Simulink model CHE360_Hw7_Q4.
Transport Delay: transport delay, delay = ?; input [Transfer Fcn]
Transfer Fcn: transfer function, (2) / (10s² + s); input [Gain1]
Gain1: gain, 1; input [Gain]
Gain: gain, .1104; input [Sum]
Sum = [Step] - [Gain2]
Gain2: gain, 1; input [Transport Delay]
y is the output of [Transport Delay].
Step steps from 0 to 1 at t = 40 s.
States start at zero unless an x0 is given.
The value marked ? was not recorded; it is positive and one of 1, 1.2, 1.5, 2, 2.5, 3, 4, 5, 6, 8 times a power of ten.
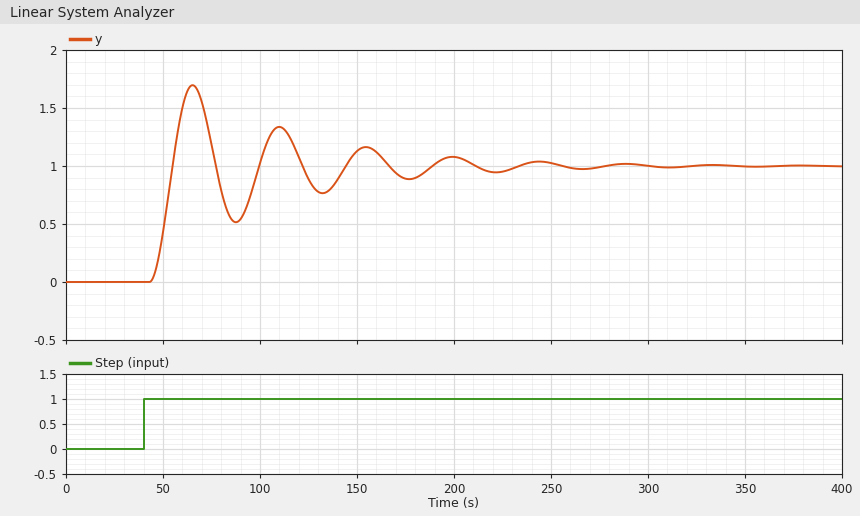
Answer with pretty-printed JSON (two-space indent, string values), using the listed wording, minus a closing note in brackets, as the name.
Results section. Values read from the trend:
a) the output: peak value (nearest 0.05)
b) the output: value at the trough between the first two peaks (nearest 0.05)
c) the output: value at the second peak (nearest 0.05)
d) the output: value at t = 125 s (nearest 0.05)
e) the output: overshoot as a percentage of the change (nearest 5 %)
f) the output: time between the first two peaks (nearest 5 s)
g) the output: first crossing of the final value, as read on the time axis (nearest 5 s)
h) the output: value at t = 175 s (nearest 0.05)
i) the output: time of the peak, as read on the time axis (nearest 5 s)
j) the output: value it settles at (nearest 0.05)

{
  "the output: peak value": "1.70",
  "the output: value at the trough between the first two peaks": "0.50",
  "the output: value at the second peak": "1.35",
  "the output: value at t = 125 s": "0.90",
  "the output: overshoot as a percentage of the change": "70 %",
  "the output: time between the first two peaks": "45 s",
  "the output: first crossing of the final value, as read on the time axis": "55 s",
  "the output: value at t = 175 s": "0.90",
  "the output: time of the peak, as read on the time axis": "65 s",
  "the output: value it settles at": "1.00"
}
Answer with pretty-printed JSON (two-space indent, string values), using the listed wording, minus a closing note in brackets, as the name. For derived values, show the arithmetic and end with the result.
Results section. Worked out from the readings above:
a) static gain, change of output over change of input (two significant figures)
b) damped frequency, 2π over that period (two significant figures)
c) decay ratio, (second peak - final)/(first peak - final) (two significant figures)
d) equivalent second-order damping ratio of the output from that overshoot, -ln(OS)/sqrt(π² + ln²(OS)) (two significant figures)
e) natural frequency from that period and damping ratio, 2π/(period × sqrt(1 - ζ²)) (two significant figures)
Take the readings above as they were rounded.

{
  "static gain, change of output over change of input": "(1 - 0) / (1 - 0) = 1.0",
  "damped frequency, 2π over that period": "2π / 45 = 0.14 rad/s",
  "decay ratio, (second peak - final)/(first peak - final)": "(1.35 - 1) / (1.7 - 1) = 0.50",
  "equivalent second-order damping ratio of the output from that overshoot, -ln(OS)/sqrt(π² + ln²(OS))": "ln(0.7) = -0.357; 0.357 / sqrt(9.870 + 0.127) = 0.11",
  "natural frequency from that period and damping ratio, 2π/(period × sqrt(1 - ζ²))": "2π / (45 × sqrt(1 - 0.11²)) = 0.14 rad/s"
}
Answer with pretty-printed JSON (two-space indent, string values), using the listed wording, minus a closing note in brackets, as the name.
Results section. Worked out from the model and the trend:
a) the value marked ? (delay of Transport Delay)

{
  "the value marked ?": "3"
}
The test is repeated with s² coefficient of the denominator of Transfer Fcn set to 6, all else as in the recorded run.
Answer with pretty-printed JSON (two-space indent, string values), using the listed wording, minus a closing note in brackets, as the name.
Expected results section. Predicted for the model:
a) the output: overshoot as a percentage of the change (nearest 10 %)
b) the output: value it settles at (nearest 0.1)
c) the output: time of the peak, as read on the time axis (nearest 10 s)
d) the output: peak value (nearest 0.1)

{
  "the output: overshoot as a percentage of the change": "60 %",
  "the output: value it settles at": "1.0",
  "the output: time of the peak, as read on the time axis": "60 s",
  "the output: peak value": "1.6"
}
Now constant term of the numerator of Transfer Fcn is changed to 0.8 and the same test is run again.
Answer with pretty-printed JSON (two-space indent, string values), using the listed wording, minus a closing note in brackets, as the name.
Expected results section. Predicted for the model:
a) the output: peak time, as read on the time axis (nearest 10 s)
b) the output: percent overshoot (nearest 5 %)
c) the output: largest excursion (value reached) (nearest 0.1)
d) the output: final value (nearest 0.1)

{
  "the output: peak time, as read on the time axis": "80 s",
  "the output: percent overshoot": "25 %",
  "the output: largest excursion (value reached)": "1.3",
  "the output: final value": "1.0"
}
